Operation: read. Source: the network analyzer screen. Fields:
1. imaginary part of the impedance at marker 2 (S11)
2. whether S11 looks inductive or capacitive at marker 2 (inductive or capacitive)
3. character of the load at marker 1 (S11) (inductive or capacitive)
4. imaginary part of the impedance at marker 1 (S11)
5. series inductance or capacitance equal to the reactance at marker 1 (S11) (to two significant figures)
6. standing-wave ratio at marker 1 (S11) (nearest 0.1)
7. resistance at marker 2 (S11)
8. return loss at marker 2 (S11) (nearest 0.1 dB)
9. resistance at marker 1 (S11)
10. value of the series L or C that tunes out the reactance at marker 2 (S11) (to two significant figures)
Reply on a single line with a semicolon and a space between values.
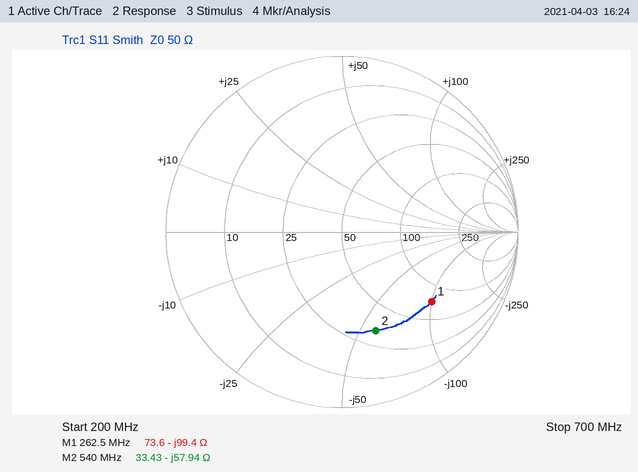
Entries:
-57.94 Ω; capacitive; capacitive; -99.4 Ω; 6.1 pF; 4.6; 33.43 Ω; 4.5 dB; 73.6 Ω; 17 nH
